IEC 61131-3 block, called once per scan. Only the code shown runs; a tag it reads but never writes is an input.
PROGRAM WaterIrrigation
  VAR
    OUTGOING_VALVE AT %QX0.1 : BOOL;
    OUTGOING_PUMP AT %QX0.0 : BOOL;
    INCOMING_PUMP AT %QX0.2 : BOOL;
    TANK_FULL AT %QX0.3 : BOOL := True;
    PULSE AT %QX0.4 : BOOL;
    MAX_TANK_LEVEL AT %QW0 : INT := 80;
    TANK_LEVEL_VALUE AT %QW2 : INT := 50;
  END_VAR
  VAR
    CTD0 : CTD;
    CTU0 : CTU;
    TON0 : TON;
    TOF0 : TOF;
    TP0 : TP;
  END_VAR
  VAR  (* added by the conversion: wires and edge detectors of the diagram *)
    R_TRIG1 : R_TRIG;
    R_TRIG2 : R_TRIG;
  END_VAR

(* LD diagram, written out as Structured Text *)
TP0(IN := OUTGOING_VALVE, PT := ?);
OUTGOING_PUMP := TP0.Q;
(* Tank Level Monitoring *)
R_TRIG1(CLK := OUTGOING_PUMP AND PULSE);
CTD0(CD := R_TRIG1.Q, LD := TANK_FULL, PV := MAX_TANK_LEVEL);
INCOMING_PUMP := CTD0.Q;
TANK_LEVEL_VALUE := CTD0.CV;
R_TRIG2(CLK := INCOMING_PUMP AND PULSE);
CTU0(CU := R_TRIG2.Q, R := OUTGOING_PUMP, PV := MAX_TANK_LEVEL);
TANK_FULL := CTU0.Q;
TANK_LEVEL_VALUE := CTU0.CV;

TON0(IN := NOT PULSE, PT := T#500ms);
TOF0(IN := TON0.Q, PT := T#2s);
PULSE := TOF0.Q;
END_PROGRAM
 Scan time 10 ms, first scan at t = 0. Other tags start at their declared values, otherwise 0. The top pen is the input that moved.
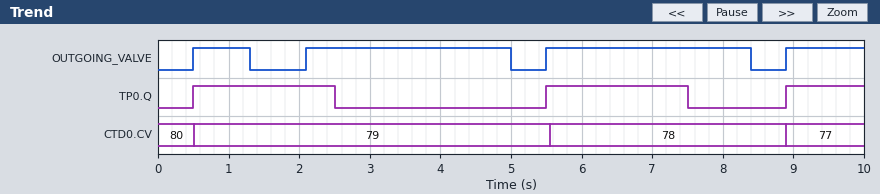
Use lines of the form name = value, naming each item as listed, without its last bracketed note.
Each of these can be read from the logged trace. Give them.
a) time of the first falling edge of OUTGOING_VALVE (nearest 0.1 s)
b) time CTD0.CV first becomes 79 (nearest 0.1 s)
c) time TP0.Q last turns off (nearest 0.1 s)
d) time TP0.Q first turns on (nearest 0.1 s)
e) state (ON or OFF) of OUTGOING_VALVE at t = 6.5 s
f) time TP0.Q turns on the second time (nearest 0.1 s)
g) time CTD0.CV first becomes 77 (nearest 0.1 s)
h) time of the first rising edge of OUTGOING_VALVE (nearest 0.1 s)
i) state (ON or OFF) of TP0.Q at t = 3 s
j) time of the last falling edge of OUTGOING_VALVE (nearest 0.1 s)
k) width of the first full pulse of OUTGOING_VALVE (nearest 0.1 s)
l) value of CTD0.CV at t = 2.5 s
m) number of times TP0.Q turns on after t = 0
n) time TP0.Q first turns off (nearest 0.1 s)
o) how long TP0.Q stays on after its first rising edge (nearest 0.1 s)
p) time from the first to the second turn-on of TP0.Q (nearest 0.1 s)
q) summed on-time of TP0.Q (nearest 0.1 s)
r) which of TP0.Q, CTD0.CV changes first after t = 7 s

time of the first falling edge of OUTGOING_VALVE = 1.3 s
time CTD0.CV first becomes 79 = 0.5 s
time TP0.Q last turns off = 7.5 s
time TP0.Q first turns on = 0.5 s
state (ON or OFF) of OUTGOING_VALVE at t = 6.5 s = ON
time TP0.Q turns on the second time = 5.5 s
time CTD0.CV first becomes 77 = 8.9 s
time of the first rising edge of OUTGOING_VALVE = 0.5 s
state (ON or OFF) of TP0.Q at t = 3 s = OFF
time of the last falling edge of OUTGOING_VALVE = 8.4 s
width of the first full pulse of OUTGOING_VALVE = 0.8 s
value of CTD0.CV at t = 2.5 s = 79
number of times TP0.Q turns on after t = 0 = 3
time TP0.Q first turns off = 2.5 s
how long TP0.Q stays on after its first rising edge = 2.0 s
time from the first to the second turn-on of TP0.Q = 5.0 s
summed on-time of TP0.Q = 5.1 s
which of TP0.Q, CTD0.CV changes first after t = 7 s = TP0.Q
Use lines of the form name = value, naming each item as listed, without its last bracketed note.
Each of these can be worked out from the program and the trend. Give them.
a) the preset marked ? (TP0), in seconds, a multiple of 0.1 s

the preset marked ? (TP0), in seconds, a multiple of 0.1 s = 2.0 s
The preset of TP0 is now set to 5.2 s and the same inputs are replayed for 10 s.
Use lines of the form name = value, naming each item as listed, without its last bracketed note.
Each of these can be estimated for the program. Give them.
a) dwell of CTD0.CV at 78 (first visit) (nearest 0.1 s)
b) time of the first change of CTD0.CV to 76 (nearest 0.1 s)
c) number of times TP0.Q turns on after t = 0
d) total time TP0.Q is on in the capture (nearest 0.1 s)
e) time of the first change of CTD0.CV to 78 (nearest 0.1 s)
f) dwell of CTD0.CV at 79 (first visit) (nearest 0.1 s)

dwell of CTD0.CV at 78 (first visit) = 2.5 s
time of the first change of CTD0.CV to 76 = 8.9 s
number of times TP0.Q turns on after t = 0 = 2
total time TP0.Q is on in the capture = 6.3 s
time of the first change of CTD0.CV to 78 = 3.0 s
dwell of CTD0.CV at 79 (first visit) = 2.5 s
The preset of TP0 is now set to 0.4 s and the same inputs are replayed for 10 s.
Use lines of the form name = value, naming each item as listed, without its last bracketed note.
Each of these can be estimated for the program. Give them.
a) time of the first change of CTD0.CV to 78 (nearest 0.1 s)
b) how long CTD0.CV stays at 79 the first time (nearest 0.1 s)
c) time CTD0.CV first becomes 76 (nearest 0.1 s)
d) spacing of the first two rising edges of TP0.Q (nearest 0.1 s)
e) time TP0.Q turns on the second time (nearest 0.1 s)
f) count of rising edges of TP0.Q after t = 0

time of the first change of CTD0.CV to 78 = 2.1 s
how long CTD0.CV stays at 79 the first time = 1.6 s
time CTD0.CV first becomes 76 = 8.9 s
spacing of the first two rising edges of TP0.Q = 1.6 s
time TP0.Q turns on the second time = 2.1 s
count of rising edges of TP0.Q after t = 0 = 4
